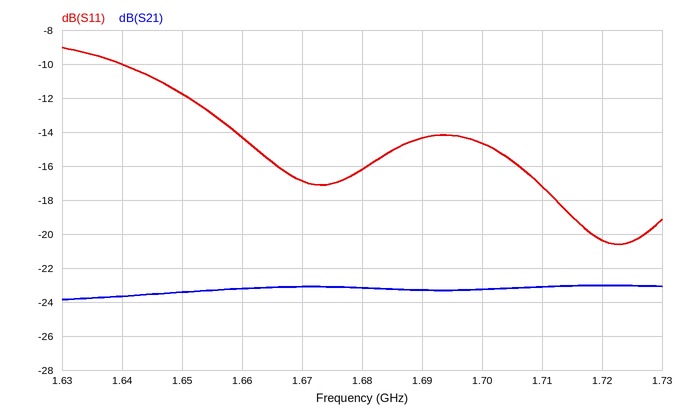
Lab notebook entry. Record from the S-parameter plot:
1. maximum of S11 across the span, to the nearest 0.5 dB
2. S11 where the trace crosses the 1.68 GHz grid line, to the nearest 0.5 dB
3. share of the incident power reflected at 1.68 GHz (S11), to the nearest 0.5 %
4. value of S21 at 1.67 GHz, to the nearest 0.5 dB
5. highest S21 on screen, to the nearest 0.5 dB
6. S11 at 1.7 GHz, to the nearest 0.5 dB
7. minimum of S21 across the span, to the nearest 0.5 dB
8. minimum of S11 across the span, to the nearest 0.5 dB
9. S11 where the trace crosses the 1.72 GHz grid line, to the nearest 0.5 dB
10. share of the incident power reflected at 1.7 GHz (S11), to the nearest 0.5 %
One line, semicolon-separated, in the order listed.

-9.0 dB; -16.0 dB; 2.5 %; -23.0 dB; -23.0 dB; -14.5 dB; -24.0 dB; -20.5 dB; -20.5 dB; 3.5 %
